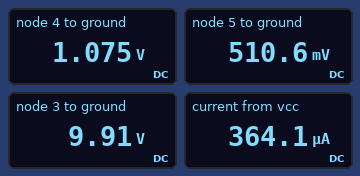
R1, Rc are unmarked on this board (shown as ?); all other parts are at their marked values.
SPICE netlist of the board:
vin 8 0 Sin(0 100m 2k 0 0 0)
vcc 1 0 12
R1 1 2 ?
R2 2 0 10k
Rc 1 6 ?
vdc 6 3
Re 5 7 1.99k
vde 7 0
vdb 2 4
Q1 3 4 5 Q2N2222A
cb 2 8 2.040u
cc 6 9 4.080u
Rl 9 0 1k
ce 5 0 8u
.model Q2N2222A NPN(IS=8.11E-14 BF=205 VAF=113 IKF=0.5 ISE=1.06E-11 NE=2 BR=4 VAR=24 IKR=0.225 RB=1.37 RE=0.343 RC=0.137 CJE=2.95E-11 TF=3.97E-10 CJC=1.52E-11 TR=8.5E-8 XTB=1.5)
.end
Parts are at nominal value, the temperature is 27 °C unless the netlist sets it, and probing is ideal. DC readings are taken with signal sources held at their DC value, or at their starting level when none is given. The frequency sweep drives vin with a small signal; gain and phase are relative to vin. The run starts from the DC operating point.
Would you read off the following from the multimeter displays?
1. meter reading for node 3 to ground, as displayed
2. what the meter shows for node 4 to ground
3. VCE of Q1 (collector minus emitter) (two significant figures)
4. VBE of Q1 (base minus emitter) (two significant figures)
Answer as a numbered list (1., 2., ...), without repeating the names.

1. 9.91 V
2. 1.075 V
3. 9.4 V
4. 560 mV
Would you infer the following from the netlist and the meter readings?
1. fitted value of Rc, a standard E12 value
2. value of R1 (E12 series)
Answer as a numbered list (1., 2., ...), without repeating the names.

1. 8.2 kΩ
2. 100 kΩ
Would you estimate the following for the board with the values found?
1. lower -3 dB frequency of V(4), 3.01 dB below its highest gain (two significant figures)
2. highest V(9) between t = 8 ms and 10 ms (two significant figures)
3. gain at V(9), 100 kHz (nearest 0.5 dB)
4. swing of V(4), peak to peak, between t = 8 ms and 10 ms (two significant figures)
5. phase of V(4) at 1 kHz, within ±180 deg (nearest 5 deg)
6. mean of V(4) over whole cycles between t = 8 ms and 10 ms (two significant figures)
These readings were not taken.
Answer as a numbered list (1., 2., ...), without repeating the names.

1. 9.0 Hz
2. 240 mV
3. 19.0 dB
4. 200 mV
5. 0 deg
6. 1.1 V
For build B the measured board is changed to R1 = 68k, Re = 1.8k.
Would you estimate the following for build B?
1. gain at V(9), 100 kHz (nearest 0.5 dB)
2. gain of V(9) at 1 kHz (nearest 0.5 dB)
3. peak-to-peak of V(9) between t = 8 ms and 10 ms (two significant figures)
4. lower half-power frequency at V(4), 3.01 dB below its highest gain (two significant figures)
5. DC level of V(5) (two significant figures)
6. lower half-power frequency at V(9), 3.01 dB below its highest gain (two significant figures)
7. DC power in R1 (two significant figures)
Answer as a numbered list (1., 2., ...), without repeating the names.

1. 25.0 dB
2. 24.0 dB
3. 2.2 V
4. 9.4 Hz
5. 930 mV
6. 410 Hz
7. 1.6 mW
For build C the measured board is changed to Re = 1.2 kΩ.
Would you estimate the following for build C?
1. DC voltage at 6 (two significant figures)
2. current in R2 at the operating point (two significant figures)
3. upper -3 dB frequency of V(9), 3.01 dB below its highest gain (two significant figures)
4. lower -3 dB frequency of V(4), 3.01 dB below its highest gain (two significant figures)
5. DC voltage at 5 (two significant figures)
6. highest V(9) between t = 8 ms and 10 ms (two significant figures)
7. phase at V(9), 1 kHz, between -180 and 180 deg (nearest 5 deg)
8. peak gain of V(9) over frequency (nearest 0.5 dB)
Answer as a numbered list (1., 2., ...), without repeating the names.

1. 8.7 V
2. 110 µA
3. 26 MHz
4. 9.1 Hz
5. 490 mV
6. 380 mV
7. -160 deg
8. 23.0 dB
